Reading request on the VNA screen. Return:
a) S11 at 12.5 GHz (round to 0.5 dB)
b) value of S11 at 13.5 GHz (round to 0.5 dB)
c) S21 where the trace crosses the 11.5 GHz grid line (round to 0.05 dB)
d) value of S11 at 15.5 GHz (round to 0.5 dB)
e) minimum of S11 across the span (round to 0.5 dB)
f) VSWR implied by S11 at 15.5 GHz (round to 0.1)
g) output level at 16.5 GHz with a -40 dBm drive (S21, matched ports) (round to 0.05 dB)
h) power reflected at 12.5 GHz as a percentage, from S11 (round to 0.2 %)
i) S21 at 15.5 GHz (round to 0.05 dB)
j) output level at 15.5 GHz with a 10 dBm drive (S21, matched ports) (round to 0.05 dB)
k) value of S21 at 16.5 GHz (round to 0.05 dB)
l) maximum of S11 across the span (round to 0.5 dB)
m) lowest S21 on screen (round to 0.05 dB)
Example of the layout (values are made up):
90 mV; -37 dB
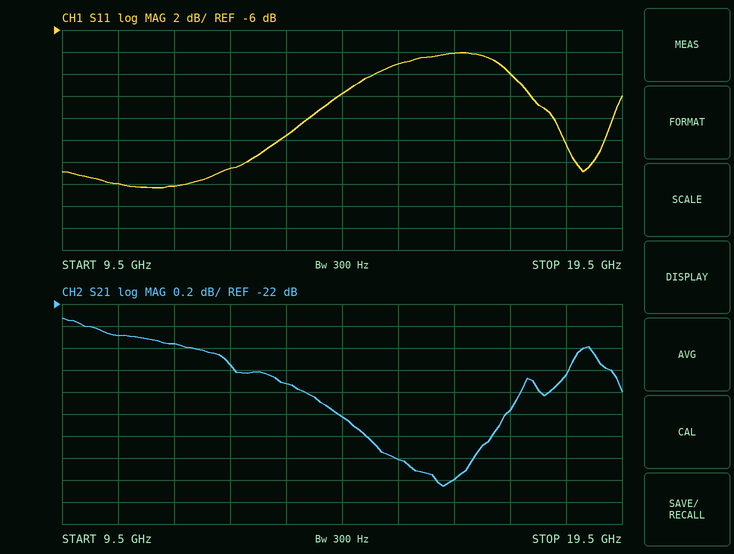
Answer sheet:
-18.5 dB; -15.5 dB; -22.35 dB; -9.0 dB; -20.5 dB; 2.1; -63.60 dBm; 1.4 %; -23.40 dB; -13.40 dBm; -23.60 dB; -8.0 dB; -23.65 dB
